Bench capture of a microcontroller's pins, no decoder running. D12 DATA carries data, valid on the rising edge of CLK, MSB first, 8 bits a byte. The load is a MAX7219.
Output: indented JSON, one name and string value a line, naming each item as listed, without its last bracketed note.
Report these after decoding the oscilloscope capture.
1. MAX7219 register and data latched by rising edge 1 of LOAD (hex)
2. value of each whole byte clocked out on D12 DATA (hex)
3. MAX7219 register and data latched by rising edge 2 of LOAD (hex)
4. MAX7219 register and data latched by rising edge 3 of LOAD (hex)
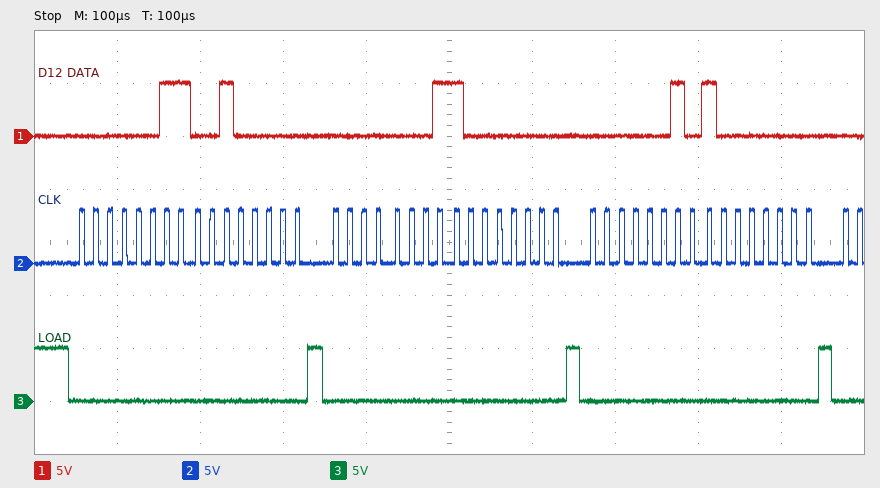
{
  "MAX7219 register and data latched by rising edge 1 of LOAD": "register 0x3, data 0x20",
  "value of each whole byte clocked out on D12 DATA": "03 20 01 80 02 80",
  "MAX7219 register and data latched by rising edge 2 of LOAD": "register 0x1, data 0x80",
  "MAX7219 register and data latched by rising edge 3 of LOAD": "register 0x2, data 0x80"
}
